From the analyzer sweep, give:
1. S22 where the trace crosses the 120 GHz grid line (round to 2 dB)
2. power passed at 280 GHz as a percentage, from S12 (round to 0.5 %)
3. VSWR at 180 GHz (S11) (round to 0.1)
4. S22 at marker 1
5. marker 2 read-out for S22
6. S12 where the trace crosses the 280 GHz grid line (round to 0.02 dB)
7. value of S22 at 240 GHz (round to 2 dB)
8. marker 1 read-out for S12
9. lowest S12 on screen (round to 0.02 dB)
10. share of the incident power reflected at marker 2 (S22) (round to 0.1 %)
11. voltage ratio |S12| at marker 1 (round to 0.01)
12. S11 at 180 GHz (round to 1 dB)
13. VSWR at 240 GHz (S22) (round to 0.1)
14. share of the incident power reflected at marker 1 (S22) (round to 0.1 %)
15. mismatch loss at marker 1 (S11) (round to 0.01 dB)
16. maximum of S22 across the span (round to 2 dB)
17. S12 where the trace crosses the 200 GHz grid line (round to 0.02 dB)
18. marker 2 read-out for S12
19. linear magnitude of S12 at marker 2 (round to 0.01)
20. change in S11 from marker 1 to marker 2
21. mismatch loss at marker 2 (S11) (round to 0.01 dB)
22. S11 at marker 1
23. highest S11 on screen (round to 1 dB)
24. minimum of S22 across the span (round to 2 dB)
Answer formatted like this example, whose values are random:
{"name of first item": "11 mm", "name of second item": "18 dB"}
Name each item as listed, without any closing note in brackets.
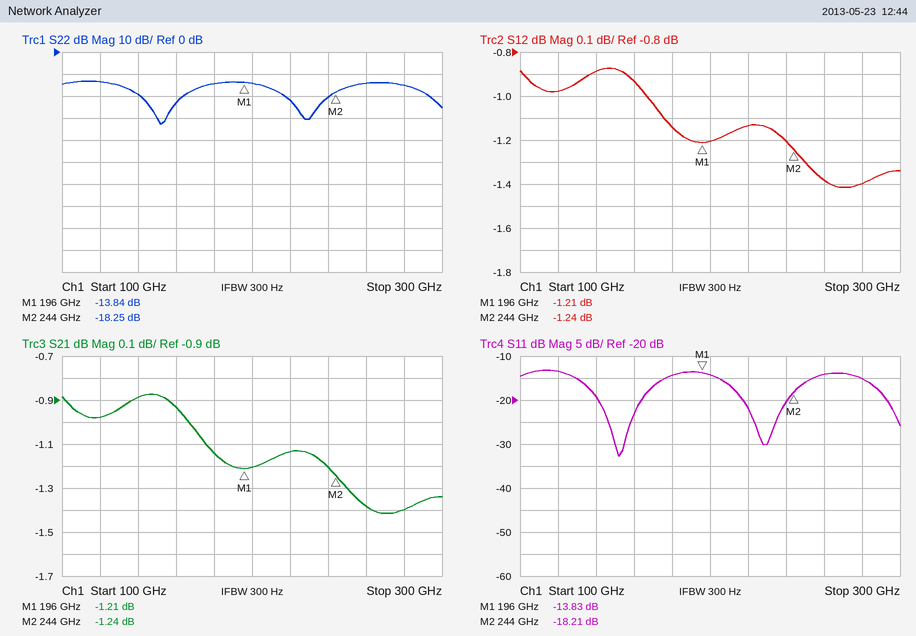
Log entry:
{"S22 where the trace crosses the 120 GHz grid line": "-14 dB", "power passed at 280 GHz as a percentage, from S12": "72.5 %", "VSWR at 180 GHz (S11)": "1.5", "S22 at marker 1": "-13.84 dB", "marker 2 read-out for S22": "-18.25 dB", "S12 where the trace crosses the 280 GHz grid line": "-1.40 dB", "value of S22 at 240 GHz": "-20 dB", "marker 1 read-out for S12": "-1.21 dB", "lowest S12 on screen": "-1.42 dB", "share of the incident power reflected at marker 2 (S22)": "1.5 %", "voltage ratio |S12| at marker 1": "0.87", "S11 at 180 GHz": "-14 dB", "VSWR at 240 GHz (S22)": "1.2", "share of the incident power reflected at marker 1 (S22)": "4.1 %", "mismatch loss at marker 1 (S11)": "0.18 dB", "maximum of S22 across the span": "-14 dB", "S12 where the trace crosses the 200 GHz grid line": "-1.20 dB", "marker 2 read-out for S12": "-1.24 dB", "linear magnitude of S12 at marker 2": "0.87", "change in S11 from marker 1 to marker 2": "-4.38 dB", "mismatch loss at marker 2 (S11)": "0.07 dB", "S11 at marker 1": "-13.83 dB", "highest S11 on screen": "-13 dB", "minimum of S22 across the span": "-32 dB"}
